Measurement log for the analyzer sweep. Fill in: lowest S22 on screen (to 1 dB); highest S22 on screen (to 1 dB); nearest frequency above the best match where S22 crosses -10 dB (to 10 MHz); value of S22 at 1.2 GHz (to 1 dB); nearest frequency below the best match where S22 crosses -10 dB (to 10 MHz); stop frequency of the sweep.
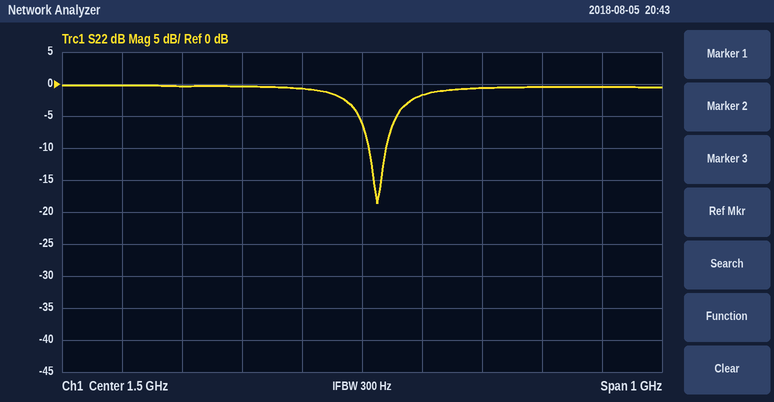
-19 dB
0 dB
1.54 GHz
0 dB
1.51 GHz
2 GHz
